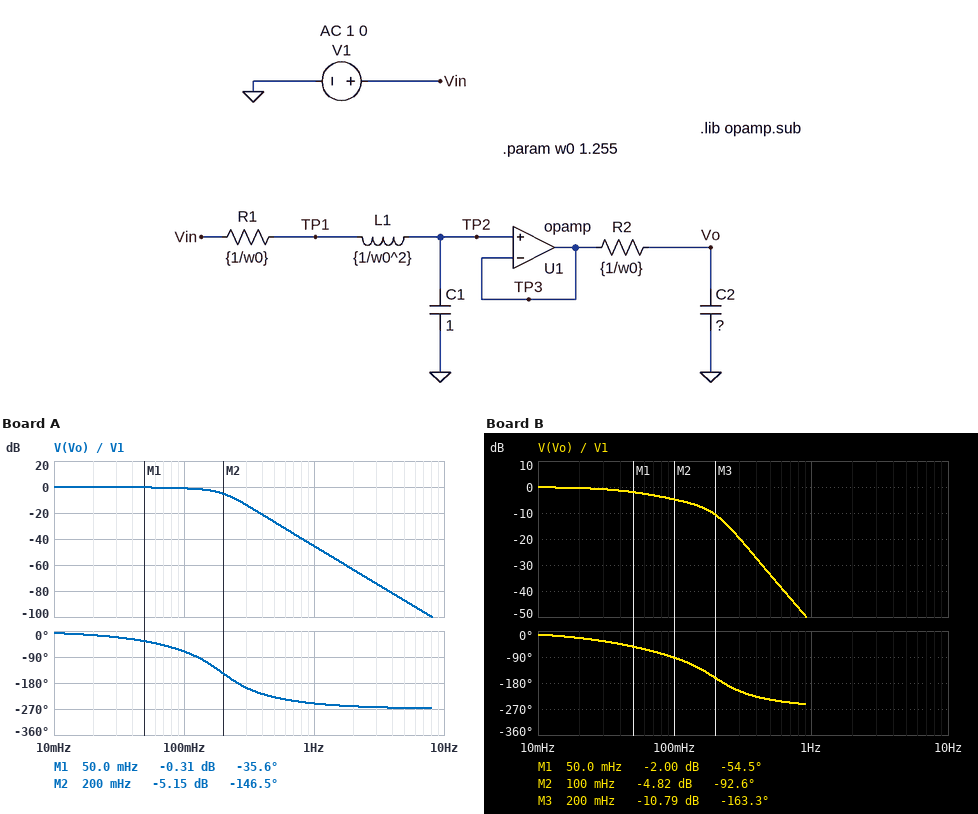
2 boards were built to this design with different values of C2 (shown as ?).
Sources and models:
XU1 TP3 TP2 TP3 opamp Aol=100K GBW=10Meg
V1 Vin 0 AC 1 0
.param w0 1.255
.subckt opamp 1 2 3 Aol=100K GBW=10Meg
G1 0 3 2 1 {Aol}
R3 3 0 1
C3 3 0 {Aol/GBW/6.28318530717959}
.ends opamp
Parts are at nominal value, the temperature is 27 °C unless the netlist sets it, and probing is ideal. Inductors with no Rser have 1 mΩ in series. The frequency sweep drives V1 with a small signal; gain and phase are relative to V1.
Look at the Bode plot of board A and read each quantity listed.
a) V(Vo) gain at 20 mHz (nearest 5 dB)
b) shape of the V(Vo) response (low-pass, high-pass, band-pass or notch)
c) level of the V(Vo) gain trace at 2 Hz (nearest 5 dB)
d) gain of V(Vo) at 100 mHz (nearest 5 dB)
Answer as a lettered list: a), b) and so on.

a) 0 dB
b) low-pass
c) -65 dB
d) 0 dB
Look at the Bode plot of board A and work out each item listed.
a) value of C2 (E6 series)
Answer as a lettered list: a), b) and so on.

a) 1.5 F
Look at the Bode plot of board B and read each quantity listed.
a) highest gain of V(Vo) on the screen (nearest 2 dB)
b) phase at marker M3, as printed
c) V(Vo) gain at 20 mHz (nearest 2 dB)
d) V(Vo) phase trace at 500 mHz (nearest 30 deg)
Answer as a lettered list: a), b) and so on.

a) 0 dB
b) -163.3 deg
c) 0 dB
d) -240 deg
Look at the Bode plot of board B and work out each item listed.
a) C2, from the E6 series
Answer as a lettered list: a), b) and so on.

a) 3.3 F
